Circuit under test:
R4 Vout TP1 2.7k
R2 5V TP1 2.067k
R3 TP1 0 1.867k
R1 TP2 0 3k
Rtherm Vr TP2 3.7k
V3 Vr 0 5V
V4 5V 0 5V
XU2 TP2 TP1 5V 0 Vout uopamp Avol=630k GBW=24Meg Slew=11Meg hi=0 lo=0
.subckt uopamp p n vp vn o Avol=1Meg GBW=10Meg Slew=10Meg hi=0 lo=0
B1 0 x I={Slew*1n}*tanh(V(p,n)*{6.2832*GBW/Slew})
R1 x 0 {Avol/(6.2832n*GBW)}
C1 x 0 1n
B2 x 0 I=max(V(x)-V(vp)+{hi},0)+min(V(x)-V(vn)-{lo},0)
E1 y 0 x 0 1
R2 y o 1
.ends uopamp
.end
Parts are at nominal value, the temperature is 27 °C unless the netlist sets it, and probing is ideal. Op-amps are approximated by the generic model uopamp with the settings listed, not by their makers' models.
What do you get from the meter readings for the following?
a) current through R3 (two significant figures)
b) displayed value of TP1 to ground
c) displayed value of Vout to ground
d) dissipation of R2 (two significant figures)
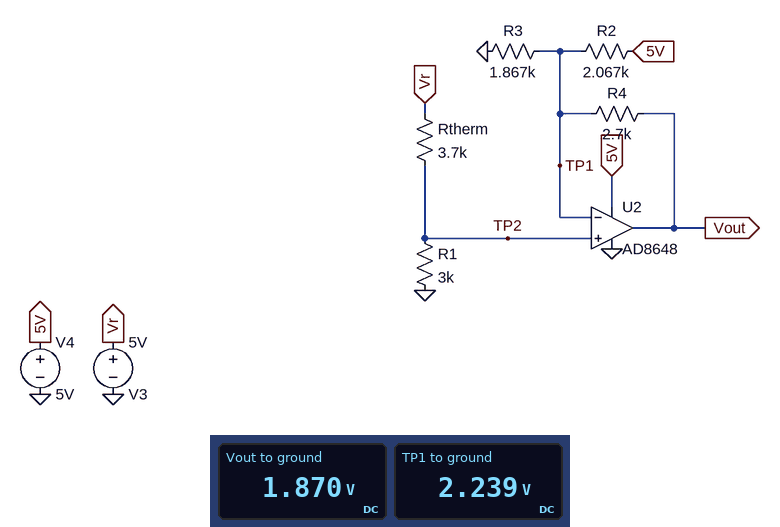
1.2 mA
2.239 V
1.870 V
3.7 mW
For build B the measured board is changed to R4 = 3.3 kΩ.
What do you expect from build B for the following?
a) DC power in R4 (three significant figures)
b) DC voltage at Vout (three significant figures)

61.7 µW
1.79 V
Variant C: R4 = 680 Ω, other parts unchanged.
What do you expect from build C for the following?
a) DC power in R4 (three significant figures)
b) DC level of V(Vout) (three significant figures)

12.7 µW
2.15 V
